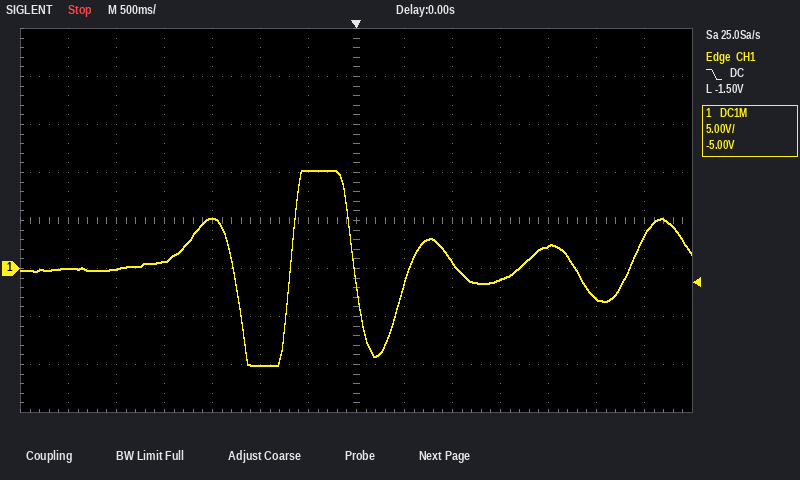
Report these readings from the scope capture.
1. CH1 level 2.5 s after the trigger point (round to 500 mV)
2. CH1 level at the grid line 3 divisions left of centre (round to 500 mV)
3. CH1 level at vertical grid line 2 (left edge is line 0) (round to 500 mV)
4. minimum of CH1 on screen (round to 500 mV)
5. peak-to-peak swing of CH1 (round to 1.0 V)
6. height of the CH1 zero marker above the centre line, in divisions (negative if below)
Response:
-3.0 V
5.0 V
0.0 V
-10.0 V
20.0 V
-1.0 div
